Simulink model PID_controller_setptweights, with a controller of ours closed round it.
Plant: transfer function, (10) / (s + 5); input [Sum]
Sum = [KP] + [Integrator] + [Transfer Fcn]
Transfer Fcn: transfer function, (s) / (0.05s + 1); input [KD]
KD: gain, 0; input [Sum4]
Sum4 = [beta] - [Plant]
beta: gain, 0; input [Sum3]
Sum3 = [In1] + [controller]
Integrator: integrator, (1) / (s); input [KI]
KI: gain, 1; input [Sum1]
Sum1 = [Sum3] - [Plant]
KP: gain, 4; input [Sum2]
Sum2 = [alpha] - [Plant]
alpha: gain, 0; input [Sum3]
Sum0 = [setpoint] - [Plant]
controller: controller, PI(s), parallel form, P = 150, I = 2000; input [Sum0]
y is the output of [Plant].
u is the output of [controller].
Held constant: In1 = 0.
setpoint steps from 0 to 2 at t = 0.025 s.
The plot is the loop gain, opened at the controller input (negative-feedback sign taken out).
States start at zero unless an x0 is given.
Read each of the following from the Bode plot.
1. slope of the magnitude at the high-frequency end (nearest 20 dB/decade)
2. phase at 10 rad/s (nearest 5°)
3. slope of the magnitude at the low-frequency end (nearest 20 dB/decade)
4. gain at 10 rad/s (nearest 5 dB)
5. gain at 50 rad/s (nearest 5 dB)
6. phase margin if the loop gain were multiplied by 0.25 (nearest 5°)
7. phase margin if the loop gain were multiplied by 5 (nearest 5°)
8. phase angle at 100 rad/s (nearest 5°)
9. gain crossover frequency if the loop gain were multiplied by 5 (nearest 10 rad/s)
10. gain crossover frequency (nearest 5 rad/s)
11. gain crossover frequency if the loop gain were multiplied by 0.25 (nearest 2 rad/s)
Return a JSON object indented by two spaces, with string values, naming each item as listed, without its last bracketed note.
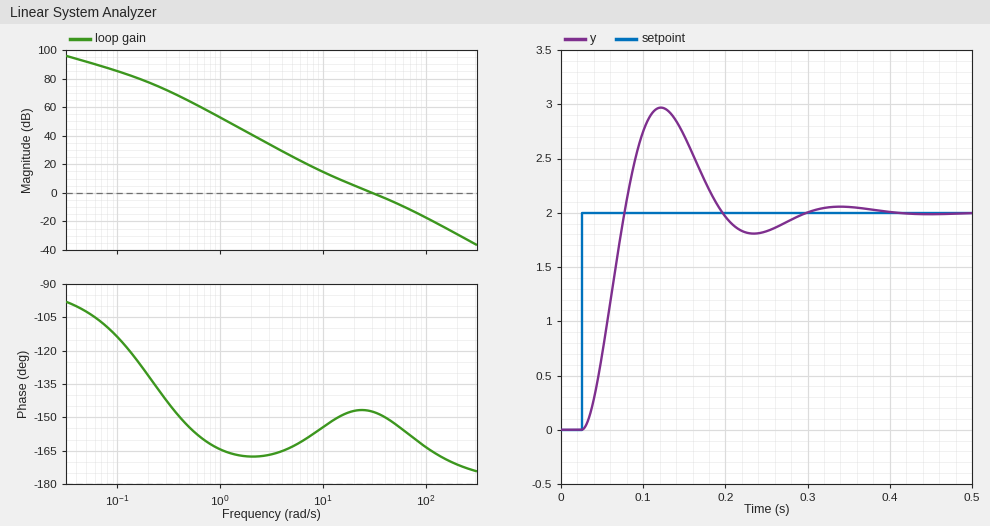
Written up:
{
  "slope of the magnitude at the high-frequency end": "-40 dB/decade",
  "phase at 10 rad/s": "-155°",
  "slope of the magnitude at the low-frequency end": "-20 dB/decade",
  "gain at 10 rad/s": "15 dB",
  "gain at 50 rad/s": "-5 dB",
  "phase margin if the loop gain were multiplied by 0.25": "30°",
  "phase margin if the loop gain were multiplied by 5": "20°",
  "phase angle at 100 rad/s": "-165°",
  "gain crossover frequency if the loop gain were multiplied by 5": "80 rad/s",
  "gain crossover frequency": "30 rad/s",
  "gain crossover frequency if the loop gain were multiplied by 0.25": "12 rad/s"
}
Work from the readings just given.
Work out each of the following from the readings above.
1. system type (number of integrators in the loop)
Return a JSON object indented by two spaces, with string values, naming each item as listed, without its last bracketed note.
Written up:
{
  "system type": "1"
}
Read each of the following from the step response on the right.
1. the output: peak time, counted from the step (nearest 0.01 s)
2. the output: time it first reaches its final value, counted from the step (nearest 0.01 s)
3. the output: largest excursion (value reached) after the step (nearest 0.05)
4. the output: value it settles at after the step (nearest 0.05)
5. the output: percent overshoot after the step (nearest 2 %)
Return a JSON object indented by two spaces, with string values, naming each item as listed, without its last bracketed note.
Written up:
{
  "the output: peak time, counted from the step": "0.10 s",
  "the output: time it first reaches its final value, counted from the step": "0.05 s",
  "the output: largest excursion (value reached) after the step": "2.95",
  "the output: value it settles at after the step": "2.00",
  "the output: percent overshoot after the step": "48 %"
}
